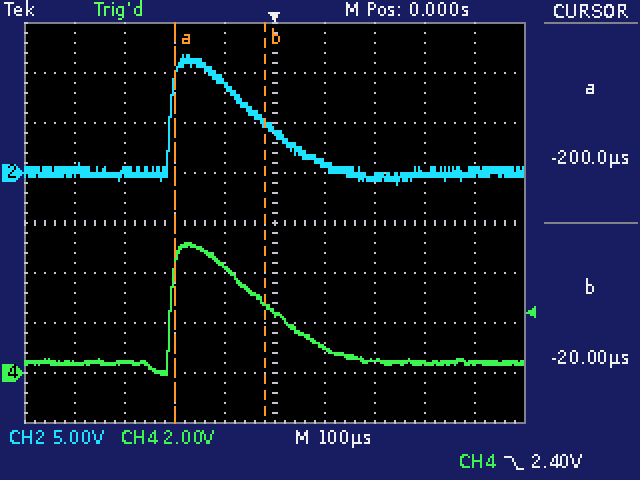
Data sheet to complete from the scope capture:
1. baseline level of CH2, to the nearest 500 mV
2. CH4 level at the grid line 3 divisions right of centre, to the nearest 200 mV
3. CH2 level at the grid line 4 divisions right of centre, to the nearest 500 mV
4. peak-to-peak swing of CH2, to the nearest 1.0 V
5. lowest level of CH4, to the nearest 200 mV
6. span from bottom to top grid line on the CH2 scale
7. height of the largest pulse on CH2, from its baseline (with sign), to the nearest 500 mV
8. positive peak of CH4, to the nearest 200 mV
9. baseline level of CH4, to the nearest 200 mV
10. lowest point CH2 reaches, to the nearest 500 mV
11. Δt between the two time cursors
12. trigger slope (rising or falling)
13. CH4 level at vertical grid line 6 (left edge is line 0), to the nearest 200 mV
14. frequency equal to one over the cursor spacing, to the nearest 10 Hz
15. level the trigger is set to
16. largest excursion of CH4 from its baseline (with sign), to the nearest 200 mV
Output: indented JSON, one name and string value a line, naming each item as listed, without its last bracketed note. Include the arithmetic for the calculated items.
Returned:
{
  "baseline level of CH2, to the nearest 500 mV": "0.0 V",
  "CH4 level at the grid line 3 divisions right of centre, to the nearest 200 mV": "400 mV",
  "CH2 level at the grid line 4 divisions right of centre, to the nearest 500 mV": "0.0 V",
  "peak-to-peak swing of CH2, to the nearest 1.0 V": "13.0 V",
  "lowest level of CH4, to the nearest 200 mV": "0.0 V",
  "span from bottom to top grid line on the CH2 scale": "40 V",
  "height of the largest pulse on CH2, from its baseline (with sign), to the nearest 500 mV": "+11.5 V",
  "positive peak of CH4, to the nearest 200 mV": "5.2 V",
  "baseline level of CH4, to the nearest 200 mV": "400 mV",
  "lowest point CH2 reaches, to the nearest 500 mV": "-1.0 V",
  "Δt between the two time cursors": "-20 µs − (-200 µs) = 180 µs",
  "trigger slope": "falling",
  "CH4 level at vertical grid line 6 (left edge is line 0), to the nearest 200 mV": "1.0 V",
  "frequency equal to one over the cursor spacing, to the nearest 10 Hz": "1 / 180 µs ≈ 5.56 kHz",
  "level the trigger is set to": "2.40 V",
  "largest excursion of CH4 from its baseline (with sign), to the nearest 200 mV": "5.2 V − (400 mV) = +4.8 V"
}
